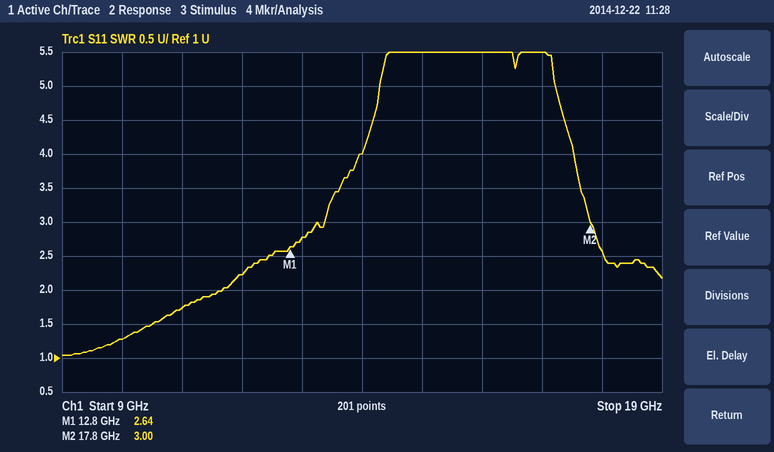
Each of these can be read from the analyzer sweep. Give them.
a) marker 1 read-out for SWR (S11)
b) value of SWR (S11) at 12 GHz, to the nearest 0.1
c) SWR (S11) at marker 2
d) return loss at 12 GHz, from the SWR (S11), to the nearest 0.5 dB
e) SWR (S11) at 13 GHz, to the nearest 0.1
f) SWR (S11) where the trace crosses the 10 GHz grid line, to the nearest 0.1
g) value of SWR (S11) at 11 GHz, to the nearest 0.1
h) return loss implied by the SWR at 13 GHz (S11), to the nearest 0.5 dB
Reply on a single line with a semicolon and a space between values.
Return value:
2.64; 2.2; 3.00; 8.5 dB; 2.8; 1.3; 1.7; 6.5 dB
